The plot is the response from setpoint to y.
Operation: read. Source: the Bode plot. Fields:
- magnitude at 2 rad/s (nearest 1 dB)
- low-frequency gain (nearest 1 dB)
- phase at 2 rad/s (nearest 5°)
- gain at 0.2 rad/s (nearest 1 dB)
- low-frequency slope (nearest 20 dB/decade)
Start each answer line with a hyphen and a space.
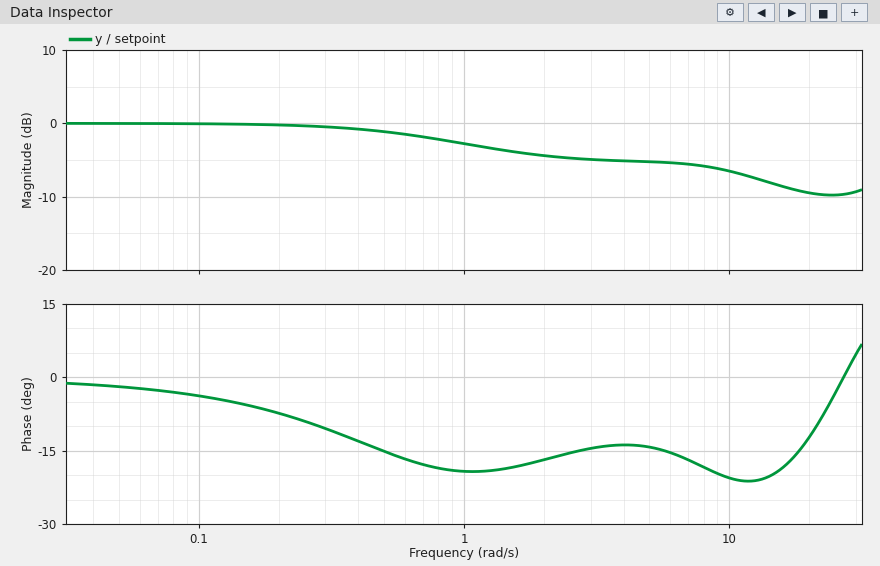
- -4 dB
- 0 dB
- -15°
- 0 dB
- 0 dB/decade
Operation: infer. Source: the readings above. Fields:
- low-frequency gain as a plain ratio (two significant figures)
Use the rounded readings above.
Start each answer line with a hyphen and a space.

- 1.0
